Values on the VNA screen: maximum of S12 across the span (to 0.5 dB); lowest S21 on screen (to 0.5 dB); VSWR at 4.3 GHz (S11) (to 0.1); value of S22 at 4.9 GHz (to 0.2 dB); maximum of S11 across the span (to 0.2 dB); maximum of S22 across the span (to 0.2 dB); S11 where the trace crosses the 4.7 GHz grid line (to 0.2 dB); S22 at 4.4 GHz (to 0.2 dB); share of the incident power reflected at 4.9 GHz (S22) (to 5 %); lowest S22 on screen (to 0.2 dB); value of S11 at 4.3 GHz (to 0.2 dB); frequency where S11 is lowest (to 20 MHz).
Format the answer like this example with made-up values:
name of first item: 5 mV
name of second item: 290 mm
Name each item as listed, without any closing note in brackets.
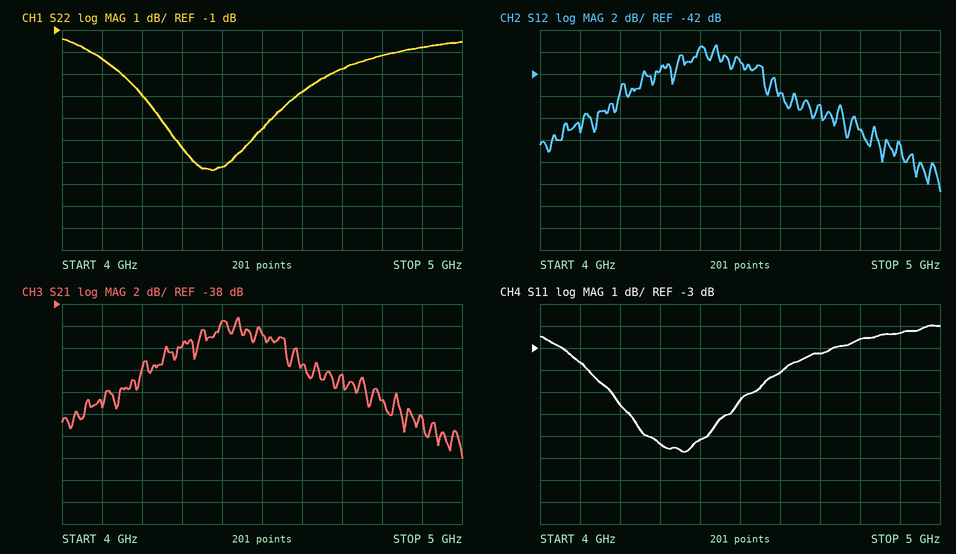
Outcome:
maximum of S12 across the span: -39.5 dB
lowest S21 on screen: -52.0 dB
VSWR at 4.3 GHz (S11): 2.5
value of S22 at 4.9 GHz: -1.8 dB
maximum of S11 across the span: -2.0 dB
maximum of S22 across the span: -1.4 dB
S11 where the trace crosses the 4.7 GHz grid line: -3.2 dB
S22 at 4.4 GHz: -7.2 dB
share of the incident power reflected at 4.9 GHz (S22): 65 %
lowest S22 on screen: -7.4 dB
value of S11 at 4.3 GHz: -7.4 dB
frequency where S11 is lowest: 4.36 GHz
